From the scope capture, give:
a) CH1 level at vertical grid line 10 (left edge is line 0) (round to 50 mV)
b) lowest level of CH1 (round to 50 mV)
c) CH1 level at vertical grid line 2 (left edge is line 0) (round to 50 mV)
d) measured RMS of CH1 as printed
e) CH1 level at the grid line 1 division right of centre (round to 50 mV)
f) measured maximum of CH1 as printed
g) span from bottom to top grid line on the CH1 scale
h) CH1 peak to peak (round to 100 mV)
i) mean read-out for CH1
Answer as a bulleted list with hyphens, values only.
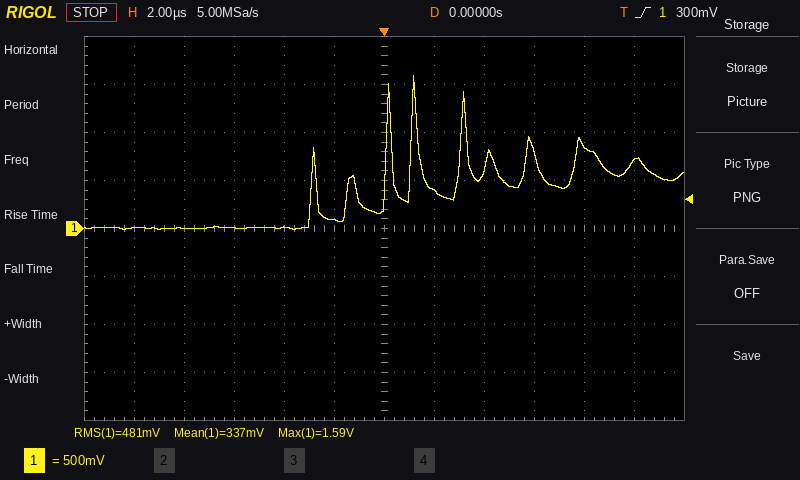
- 850 mV
- 0 mV
- 0 mV
- 481 mV
- 400 mV
- 1.59 V
- 4 V
- 1.60 V
- 337 mV
